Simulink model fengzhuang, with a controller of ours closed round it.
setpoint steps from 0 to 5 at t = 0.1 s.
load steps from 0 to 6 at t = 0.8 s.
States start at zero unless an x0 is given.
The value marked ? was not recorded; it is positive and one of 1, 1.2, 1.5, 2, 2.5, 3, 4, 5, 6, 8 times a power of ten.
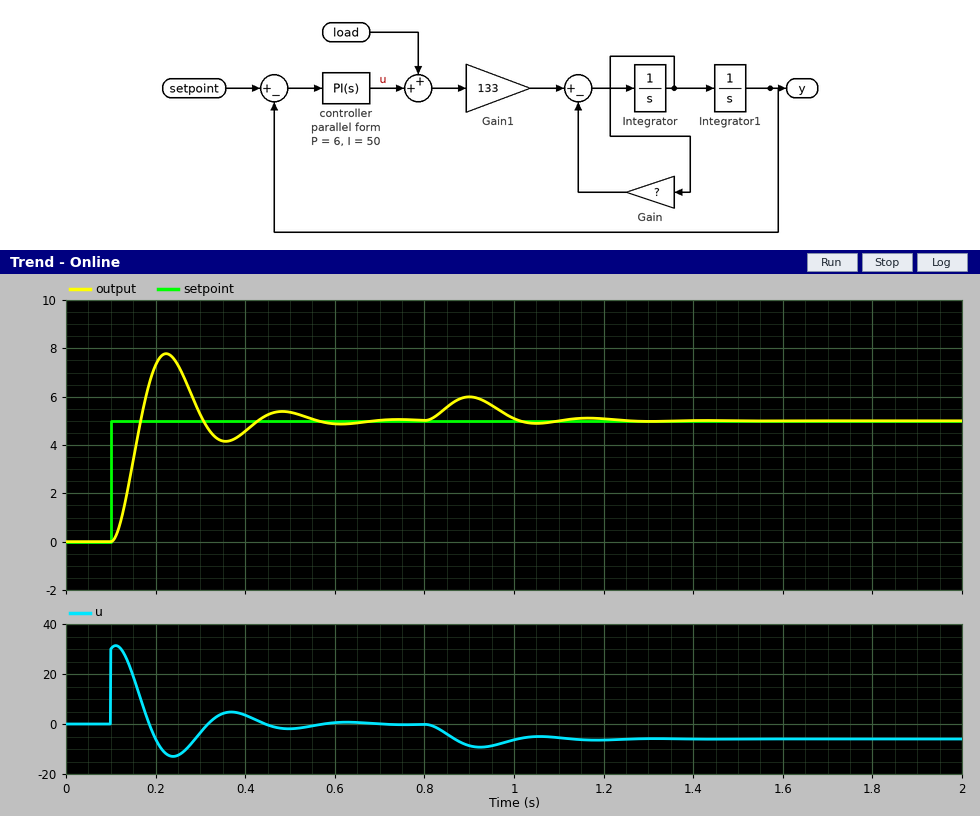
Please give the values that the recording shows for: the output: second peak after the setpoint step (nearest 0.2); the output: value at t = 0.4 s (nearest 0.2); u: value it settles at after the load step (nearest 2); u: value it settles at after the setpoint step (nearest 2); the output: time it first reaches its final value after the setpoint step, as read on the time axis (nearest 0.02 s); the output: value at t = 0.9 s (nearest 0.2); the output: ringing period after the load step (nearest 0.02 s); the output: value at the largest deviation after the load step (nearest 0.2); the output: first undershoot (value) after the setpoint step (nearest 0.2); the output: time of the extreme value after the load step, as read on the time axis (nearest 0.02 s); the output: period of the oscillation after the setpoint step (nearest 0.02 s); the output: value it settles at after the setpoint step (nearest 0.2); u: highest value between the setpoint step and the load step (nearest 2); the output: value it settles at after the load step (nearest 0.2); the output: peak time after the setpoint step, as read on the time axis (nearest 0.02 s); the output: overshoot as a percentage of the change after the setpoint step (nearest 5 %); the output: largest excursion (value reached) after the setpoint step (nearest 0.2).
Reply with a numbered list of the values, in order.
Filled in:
1. 5.4
2. 4.6
3. -6
4. 0
5. 0.16 s
6. 6.0
7. 0.26 s
8. 6.0
9. 4.2
10. 0.90 s
11. 0.26 s
12. 5.0
13. 32
14. 5.0
15. 0.22 s
16. 55 %
17. 7.8
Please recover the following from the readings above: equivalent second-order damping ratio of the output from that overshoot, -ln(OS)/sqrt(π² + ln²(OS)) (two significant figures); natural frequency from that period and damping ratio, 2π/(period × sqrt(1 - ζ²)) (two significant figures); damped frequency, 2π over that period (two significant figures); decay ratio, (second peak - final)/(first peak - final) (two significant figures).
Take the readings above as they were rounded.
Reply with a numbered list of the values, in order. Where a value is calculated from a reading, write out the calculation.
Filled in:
1. ln(0.55) = -0.598; 0.598 / sqrt(9.870 + 0.357) = 0.19
2. 2π / (0.26 × sqrt(1 - 0.19²)) = 25 rad/s
3. 2π / 0.26 = 24 rad/s
4. (5.4 - 5) / (7.8 - 5) = 0.14
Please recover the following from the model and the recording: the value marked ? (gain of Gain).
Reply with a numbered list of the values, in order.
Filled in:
1. 25
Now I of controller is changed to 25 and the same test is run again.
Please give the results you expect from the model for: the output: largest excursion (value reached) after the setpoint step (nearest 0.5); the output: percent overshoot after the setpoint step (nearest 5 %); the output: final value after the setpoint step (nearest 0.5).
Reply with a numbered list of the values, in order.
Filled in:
1. 7.0
2. 40 %
3. 5.0
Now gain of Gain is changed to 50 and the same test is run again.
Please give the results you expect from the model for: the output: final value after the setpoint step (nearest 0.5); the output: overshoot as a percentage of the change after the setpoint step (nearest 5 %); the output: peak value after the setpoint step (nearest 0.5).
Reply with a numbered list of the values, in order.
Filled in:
1. 5.0
2. 35 %
3. 6.5
